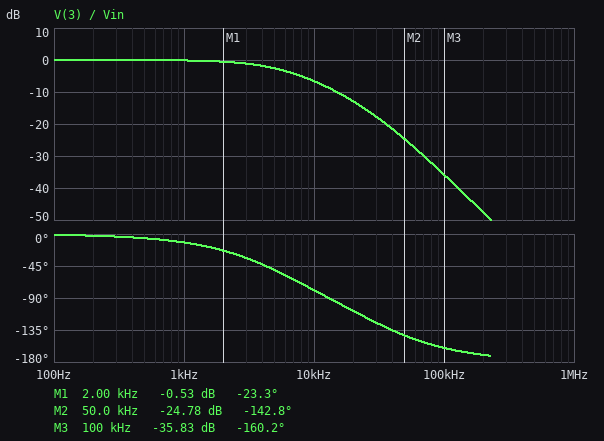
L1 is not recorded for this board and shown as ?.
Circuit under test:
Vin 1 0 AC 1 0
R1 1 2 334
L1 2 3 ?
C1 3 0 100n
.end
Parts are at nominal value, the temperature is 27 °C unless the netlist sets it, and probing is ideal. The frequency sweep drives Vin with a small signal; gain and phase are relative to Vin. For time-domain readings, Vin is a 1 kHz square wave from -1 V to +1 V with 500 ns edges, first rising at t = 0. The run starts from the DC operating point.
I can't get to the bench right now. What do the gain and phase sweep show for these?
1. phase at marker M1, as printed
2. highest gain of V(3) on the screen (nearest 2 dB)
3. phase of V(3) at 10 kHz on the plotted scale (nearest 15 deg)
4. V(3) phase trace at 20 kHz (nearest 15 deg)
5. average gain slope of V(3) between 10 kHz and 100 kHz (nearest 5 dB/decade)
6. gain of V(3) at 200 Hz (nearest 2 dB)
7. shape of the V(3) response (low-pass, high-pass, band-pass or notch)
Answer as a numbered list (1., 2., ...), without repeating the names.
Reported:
1. -23.3 deg
2. 0 dB
3. -75 deg
4. -105 deg
5. -30 dB/decade
6. 0 dB
7. low-pass
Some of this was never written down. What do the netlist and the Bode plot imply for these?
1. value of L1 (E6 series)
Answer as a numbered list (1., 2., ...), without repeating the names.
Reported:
1. 1.5 mH
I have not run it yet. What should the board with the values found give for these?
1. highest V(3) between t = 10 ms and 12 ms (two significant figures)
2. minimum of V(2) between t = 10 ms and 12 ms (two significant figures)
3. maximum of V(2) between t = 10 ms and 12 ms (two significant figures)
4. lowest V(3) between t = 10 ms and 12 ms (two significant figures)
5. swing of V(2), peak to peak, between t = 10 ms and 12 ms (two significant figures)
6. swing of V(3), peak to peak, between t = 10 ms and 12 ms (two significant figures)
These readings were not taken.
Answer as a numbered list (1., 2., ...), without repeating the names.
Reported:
1. 1.0 V
2. -1.0 V
3. 1.0 V
4. -1.0 V
5. 2.0 V
6. 2.0 V
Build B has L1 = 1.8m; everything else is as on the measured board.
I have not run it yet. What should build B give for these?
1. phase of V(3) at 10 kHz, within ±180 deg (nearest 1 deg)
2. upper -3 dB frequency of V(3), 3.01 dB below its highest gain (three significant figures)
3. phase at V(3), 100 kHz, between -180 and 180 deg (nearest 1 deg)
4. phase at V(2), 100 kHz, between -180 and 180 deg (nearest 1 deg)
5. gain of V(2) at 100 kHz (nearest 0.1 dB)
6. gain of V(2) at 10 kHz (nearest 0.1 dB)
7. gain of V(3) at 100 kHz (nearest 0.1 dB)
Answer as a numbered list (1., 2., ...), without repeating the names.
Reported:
1. -82 deg
2. 5.64 kHz
3. -163 deg
4. 17 deg
5. -0.4 dB
6. -17.3 dB
7. -37.3 dB
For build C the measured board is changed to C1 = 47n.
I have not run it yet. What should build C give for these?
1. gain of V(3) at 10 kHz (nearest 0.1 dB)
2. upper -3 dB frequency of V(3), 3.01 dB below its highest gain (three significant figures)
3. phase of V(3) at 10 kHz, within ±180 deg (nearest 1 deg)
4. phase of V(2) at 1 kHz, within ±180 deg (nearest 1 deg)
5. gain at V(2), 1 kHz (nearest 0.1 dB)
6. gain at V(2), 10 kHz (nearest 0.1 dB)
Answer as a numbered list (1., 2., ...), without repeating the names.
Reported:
1. -1.7 dB
2. 13.4 kHz
3. -54 deg
4. -6 deg
5. 0 dB
6. -4.6 dB
